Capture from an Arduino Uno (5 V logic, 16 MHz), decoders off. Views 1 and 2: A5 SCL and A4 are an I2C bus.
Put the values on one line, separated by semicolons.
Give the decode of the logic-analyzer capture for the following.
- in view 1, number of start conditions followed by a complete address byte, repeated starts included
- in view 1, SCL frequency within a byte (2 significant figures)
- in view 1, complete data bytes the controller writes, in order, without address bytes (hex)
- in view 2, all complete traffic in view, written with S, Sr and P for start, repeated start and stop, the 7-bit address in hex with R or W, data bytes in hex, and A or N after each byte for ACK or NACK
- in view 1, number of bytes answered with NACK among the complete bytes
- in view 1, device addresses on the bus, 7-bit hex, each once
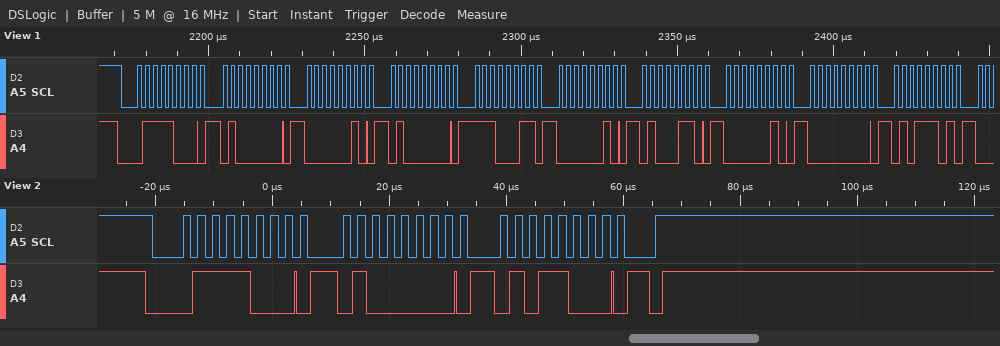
1; 400 kHz; 40 02 40 E3 02 46 02 00 5D; S 3CW A 40 A 58 A P; 0; 0x3C
